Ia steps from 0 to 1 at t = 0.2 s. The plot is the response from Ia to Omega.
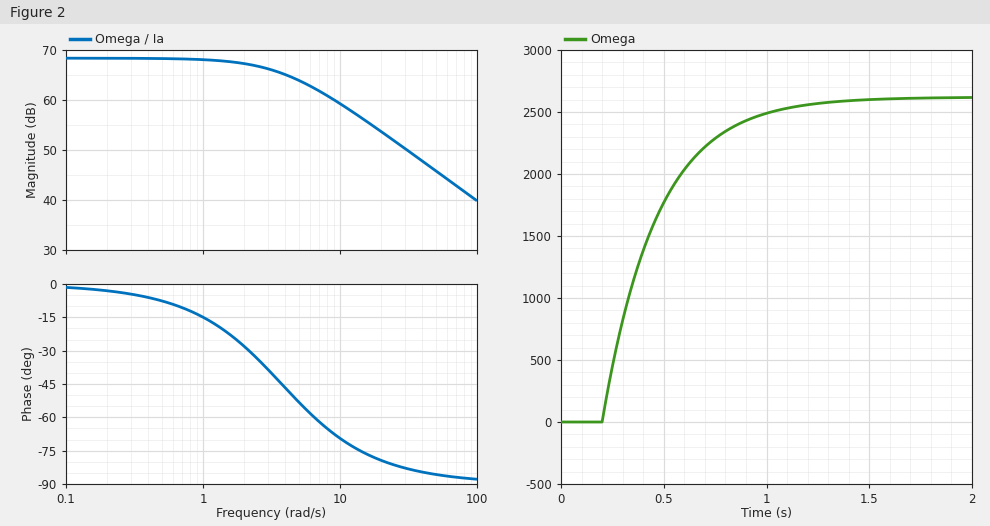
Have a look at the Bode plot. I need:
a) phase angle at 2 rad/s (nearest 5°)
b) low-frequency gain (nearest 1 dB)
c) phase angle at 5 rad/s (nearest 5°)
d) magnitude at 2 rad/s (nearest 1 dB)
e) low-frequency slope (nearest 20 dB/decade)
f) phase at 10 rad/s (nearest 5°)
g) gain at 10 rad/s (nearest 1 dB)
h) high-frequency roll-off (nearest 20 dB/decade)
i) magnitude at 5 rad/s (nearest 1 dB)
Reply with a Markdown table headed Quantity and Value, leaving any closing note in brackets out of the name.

| Quantity | Value |
|---|---|
| phase angle at 2 rad/s | -30° |
| low-frequency gain | 68 dB |
| phase angle at 5 rad/s | -55° |
| magnitude at 2 rad/s | 67 dB |
| low-frequency slope | 0 dB/decade |
| phase at 10 rad/s | -70° |
| gain at 10 rad/s | 59 dB |
| high-frequency roll-off | -20 dB/decade |
| magnitude at 5 rad/s | 64 dB |
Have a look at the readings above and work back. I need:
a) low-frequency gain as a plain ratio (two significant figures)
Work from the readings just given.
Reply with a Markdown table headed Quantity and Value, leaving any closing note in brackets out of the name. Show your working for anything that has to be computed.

| Quantity | Value |
|---|---|
| low-frequency gain as a plain ratio | 10^(68 / 20) = 2500 |
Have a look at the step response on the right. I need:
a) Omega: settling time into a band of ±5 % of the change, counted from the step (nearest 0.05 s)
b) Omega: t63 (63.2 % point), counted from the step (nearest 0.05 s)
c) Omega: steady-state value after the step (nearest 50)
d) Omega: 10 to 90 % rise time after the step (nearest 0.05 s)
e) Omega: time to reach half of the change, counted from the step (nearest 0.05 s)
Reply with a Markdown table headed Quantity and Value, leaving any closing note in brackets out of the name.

| Quantity | Value |
|---|---|
| Omega: settling time into a band of ±5 % of the change, counted from the step | 0.80 s |
| Omega: t63 (63.2 % point), counted from the step | 0.25 s |
| Omega: steady-state value after the step | 2600 |
| Omega: 10 to 90 % rise time after the step | 0.60 s |
| Omega: time to reach half of the change, counted from the step | 0.20 s |
